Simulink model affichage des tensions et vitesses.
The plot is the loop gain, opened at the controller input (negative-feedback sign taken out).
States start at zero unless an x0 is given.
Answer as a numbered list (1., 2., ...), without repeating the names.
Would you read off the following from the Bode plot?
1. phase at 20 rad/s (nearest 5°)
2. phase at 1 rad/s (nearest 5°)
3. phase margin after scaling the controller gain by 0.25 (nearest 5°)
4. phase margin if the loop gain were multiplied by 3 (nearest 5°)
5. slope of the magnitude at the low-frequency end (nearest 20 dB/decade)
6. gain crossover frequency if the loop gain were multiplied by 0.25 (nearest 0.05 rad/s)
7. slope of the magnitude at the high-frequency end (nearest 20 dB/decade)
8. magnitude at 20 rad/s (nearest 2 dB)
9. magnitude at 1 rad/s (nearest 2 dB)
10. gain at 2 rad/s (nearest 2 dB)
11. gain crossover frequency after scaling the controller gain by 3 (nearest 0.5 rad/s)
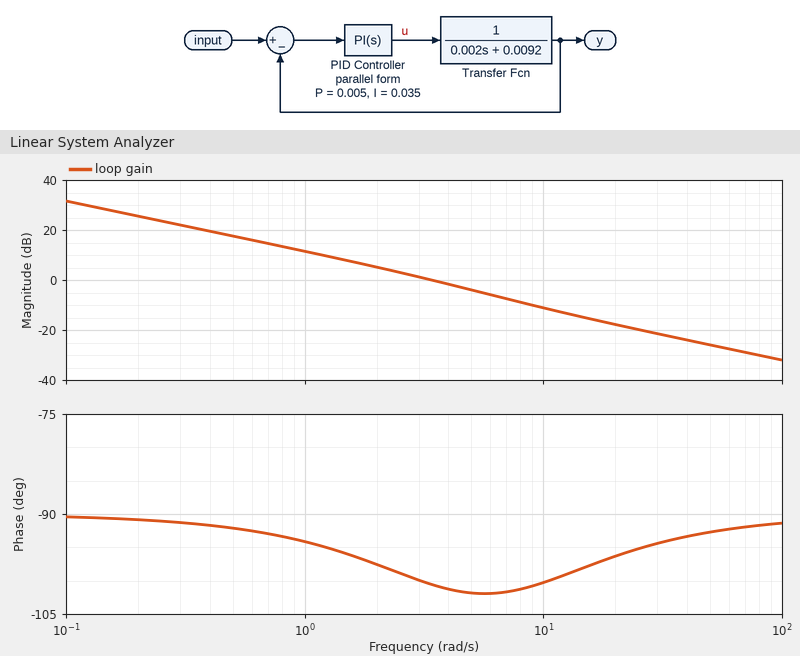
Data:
1. -95°
2. -95°
3. 85°
4. 80°
5. -20 dB/decade
6. 0.95 rad/s
7. -20 dB/decade
8. -18 dB
9. 12 dB
10. 6 dB
11. 8.5 rad/s
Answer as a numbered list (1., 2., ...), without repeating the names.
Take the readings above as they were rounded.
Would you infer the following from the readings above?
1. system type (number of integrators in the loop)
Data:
1. 1
